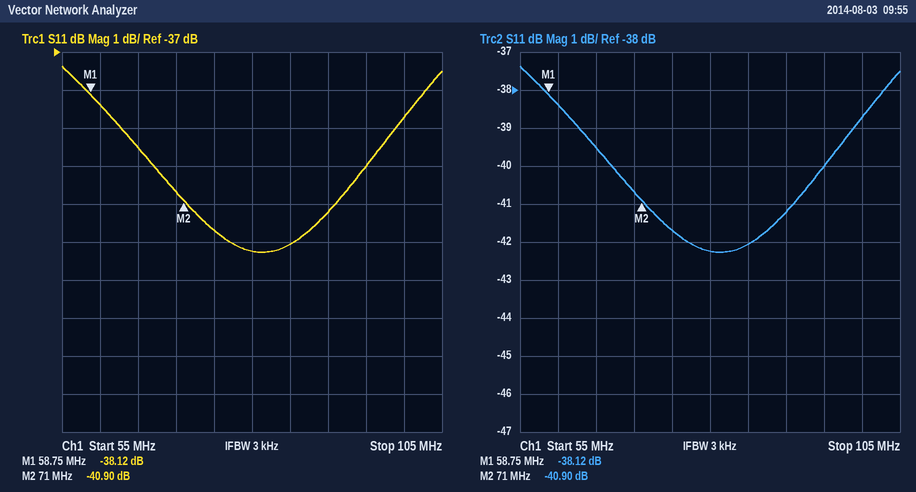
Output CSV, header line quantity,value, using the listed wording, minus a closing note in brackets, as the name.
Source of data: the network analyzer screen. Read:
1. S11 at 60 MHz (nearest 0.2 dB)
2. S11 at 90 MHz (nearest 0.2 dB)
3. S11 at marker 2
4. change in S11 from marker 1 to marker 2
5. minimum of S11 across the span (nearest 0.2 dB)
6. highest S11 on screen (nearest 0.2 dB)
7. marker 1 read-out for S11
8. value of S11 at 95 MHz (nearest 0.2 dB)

quantity,value
S11 at 60 MHz,-38.4 dB
S11 at 90 MHz,-41.2 dB
S11 at marker 2,-40.90 dB
change in S11 from marker 1 to marker 2,-2.78 dB
minimum of S11 across the span,-42.2 dB
highest S11 on screen,-37.4 dB
marker 1 read-out for S11,-38.12 dB
value of S11 at 95 MHz,-40.0 dB
